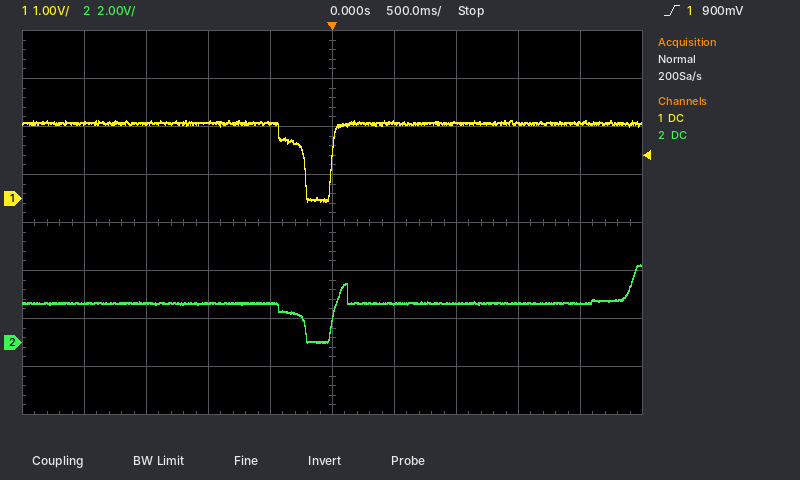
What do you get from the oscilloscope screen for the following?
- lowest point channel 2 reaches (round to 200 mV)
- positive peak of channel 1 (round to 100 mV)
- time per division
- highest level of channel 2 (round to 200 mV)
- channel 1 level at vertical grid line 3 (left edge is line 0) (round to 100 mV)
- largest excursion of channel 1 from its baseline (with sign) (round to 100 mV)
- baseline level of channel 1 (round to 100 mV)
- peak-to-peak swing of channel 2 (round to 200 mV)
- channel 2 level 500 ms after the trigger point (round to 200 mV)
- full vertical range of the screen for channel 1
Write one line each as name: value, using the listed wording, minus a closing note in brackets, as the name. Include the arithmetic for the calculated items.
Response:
lowest point channel 2 reaches: 0.0 V
positive peak of channel 1: 1.6 V
time per division: 500 ms
highest level of channel 2: 3.2 V
channel 1 level at vertical grid line 3 (left edge is line 0): 1.6 V
largest excursion of channel 1 from its baseline (with sign): -1.6 V
baseline level of channel 1: 1.6 V
peak-to-peak swing of channel 2: 3.2 V − (0.0 V) = 3.2 V
channel 2 level 500 ms after the trigger point: 1.6 V
full vertical range of the screen for channel 1: 8 V
